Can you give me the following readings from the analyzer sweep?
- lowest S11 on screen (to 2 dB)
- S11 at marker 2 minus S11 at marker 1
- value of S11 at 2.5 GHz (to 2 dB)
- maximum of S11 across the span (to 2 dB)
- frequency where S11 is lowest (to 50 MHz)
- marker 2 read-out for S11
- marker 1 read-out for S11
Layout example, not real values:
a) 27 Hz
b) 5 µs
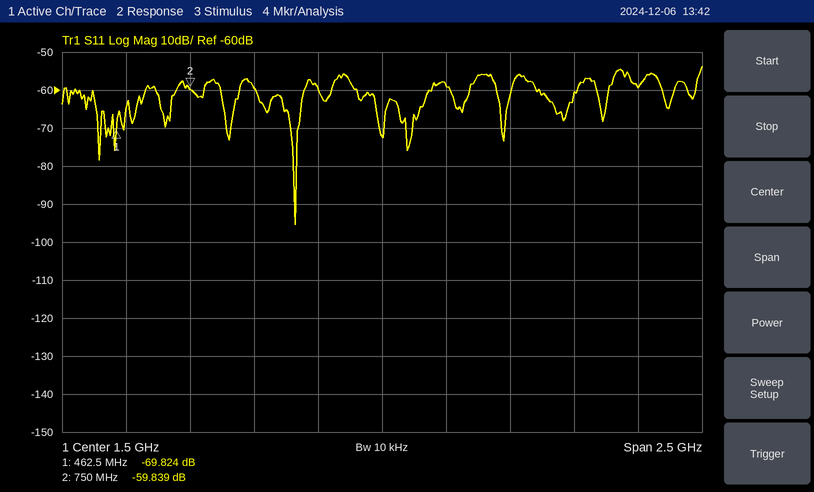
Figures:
a) -96 dB
b) 9.985 dB
c) -60 dB
d) -54 dB
e) 1.15 GHz
f) -59.839 dB
g) -69.824 dB
